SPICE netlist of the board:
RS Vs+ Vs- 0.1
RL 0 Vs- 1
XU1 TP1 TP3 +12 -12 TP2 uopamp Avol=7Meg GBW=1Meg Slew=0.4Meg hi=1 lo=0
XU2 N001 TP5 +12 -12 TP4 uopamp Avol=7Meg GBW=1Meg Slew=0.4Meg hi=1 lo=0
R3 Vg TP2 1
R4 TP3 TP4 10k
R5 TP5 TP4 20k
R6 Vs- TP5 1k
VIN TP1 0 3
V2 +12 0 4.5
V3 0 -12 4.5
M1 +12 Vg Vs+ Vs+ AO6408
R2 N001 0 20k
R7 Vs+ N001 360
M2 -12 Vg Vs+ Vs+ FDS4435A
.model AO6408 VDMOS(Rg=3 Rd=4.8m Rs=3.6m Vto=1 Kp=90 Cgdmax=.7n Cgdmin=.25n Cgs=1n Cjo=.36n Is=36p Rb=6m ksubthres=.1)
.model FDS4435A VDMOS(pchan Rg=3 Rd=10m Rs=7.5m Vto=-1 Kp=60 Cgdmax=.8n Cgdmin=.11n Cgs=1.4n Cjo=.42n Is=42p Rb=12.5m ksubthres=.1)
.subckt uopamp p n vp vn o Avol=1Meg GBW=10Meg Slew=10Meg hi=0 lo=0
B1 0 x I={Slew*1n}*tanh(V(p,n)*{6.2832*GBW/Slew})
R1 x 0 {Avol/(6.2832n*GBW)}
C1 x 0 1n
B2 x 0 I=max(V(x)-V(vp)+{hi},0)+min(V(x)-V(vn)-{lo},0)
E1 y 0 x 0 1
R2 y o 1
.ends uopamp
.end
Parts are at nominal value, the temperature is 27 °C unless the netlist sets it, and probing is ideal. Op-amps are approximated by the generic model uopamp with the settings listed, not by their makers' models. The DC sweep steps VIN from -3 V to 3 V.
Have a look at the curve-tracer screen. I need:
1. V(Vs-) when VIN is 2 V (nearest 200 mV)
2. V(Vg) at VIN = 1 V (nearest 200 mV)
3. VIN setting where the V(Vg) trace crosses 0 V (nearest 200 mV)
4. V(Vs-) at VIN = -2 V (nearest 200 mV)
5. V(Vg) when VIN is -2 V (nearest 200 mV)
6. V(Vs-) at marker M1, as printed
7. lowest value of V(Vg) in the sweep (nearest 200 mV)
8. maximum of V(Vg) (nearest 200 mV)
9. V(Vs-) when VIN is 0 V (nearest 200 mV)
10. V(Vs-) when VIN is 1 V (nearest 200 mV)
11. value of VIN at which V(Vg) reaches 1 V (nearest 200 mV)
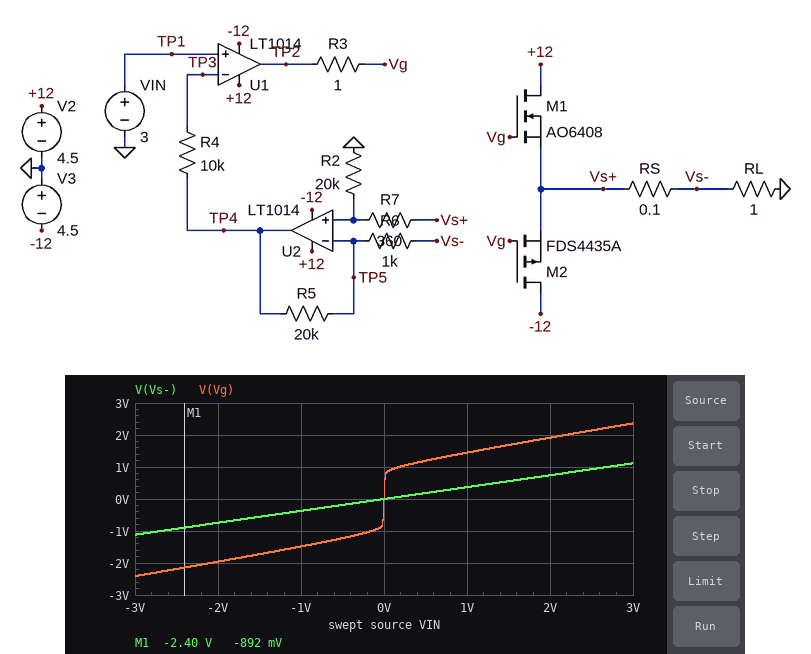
800 mV
1.4 V
0 V
-800 mV
-2.0 V
-892 mV
-2.4 V
2.4 V
0 V
400 mV
200 mV
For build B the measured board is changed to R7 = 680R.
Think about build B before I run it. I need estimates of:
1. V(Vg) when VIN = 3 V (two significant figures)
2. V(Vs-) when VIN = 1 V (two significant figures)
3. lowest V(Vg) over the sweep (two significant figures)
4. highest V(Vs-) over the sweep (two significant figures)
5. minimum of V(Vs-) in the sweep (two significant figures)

2.6 V
430 mV
-2.6 V
1.3 V
-1.3 V
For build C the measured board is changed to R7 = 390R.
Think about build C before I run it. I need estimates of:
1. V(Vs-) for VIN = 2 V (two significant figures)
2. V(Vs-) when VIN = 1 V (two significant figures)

750 mV
380 mV
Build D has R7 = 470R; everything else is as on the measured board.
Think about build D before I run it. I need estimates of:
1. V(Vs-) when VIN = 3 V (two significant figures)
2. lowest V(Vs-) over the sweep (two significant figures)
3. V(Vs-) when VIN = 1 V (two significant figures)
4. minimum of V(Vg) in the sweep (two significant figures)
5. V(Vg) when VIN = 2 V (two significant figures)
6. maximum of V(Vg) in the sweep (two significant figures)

1.2 V
-1.2 V
390 mV
-2.5 V
2.0 V
2.4 V
